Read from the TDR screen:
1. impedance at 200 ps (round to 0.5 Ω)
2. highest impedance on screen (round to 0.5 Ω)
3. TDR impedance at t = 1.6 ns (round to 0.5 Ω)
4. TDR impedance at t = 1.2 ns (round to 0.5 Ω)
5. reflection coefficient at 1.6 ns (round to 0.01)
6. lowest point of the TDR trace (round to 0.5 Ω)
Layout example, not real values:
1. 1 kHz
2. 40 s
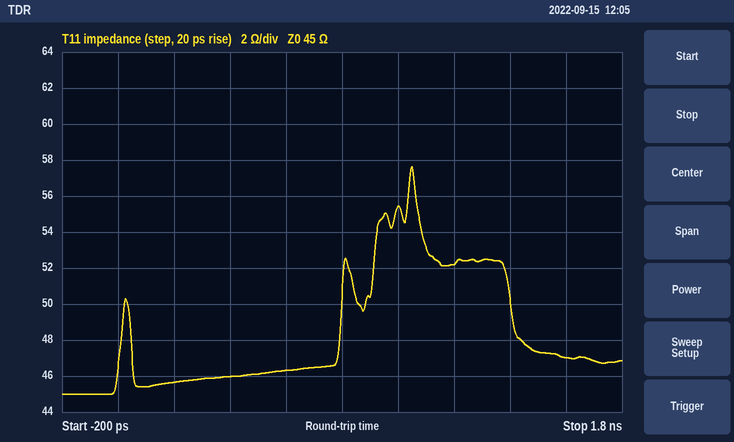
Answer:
1. 45.5 Ω
2. 57.5 Ω
3. 47.0 Ω
4. 52.0 Ω
5. +0.02
6. 45.0 Ω
